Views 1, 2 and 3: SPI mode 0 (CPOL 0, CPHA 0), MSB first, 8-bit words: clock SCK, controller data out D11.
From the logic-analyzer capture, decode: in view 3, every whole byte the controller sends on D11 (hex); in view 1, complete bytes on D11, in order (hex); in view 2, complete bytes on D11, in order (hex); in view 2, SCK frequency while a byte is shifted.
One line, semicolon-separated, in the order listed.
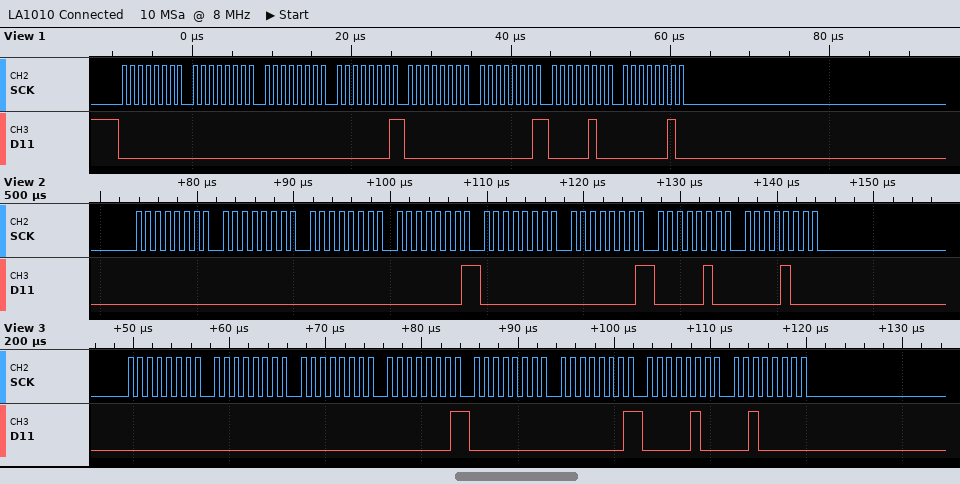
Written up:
00 00 00 01 00 01 04 20; 00 00 00 01 00 01 04 02; 0x00 0x00 0x00 0x01 0x00 0x01 0x04 0x08; 1 MHz
